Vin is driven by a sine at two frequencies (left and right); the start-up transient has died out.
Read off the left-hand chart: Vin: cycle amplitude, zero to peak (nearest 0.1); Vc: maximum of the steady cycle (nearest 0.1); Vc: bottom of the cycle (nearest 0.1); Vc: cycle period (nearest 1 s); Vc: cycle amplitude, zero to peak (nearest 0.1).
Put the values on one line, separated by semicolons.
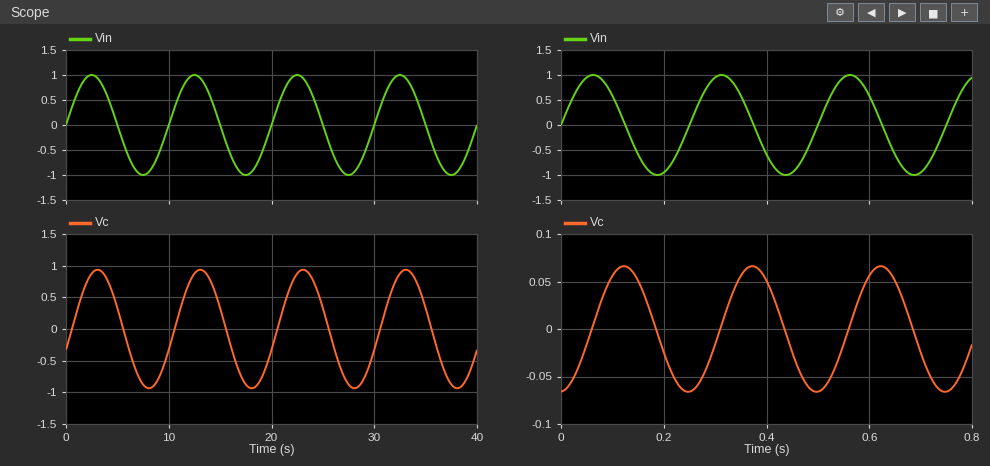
1.0; 0.9; -0.9; 10 s; 0.9
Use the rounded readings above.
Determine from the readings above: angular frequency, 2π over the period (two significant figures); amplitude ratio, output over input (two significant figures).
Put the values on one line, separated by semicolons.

0.63 rad/s; 0.90
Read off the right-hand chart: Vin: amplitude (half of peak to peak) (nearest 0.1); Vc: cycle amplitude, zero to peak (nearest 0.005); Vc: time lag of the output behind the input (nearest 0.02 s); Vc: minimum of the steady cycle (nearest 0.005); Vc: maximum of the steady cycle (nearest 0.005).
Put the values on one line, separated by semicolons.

1.0; 0.065; 0.06 s; -0.065; 0.065
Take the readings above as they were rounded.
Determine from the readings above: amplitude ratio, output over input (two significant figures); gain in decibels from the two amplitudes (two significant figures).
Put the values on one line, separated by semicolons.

0.065; -24 dB
